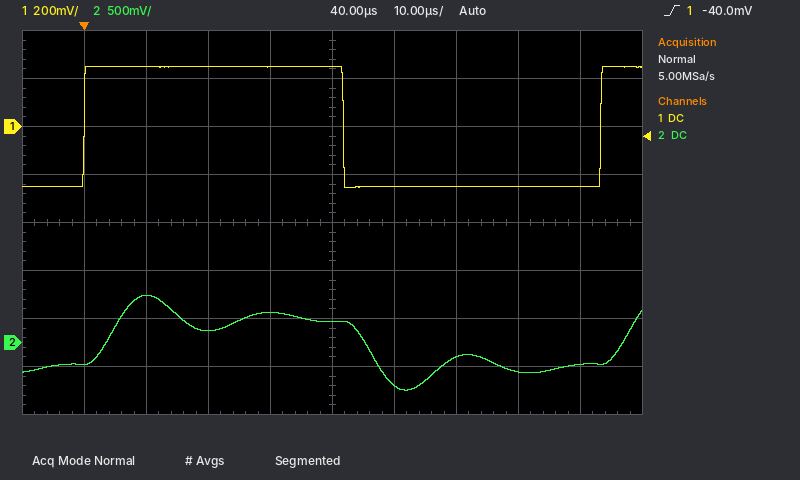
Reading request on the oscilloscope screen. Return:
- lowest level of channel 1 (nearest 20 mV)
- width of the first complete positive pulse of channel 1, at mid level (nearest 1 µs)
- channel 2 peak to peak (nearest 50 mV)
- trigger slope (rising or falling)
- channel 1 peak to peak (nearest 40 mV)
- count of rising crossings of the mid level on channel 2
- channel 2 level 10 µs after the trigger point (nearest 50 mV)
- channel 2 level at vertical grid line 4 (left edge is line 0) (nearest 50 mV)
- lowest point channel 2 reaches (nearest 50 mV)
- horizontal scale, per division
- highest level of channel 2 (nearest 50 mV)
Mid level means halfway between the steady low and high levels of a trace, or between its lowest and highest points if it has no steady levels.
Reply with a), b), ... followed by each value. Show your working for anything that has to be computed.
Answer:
a) -260 mV
b) 42 µs
c) 500 mV − (-500 mV) = 1.00 V
d) rising
e) 520 mV
f) 2
g) 500 mV
h) 300 mV
i) -500 mV
j) 10 µs
k) 500 mV
